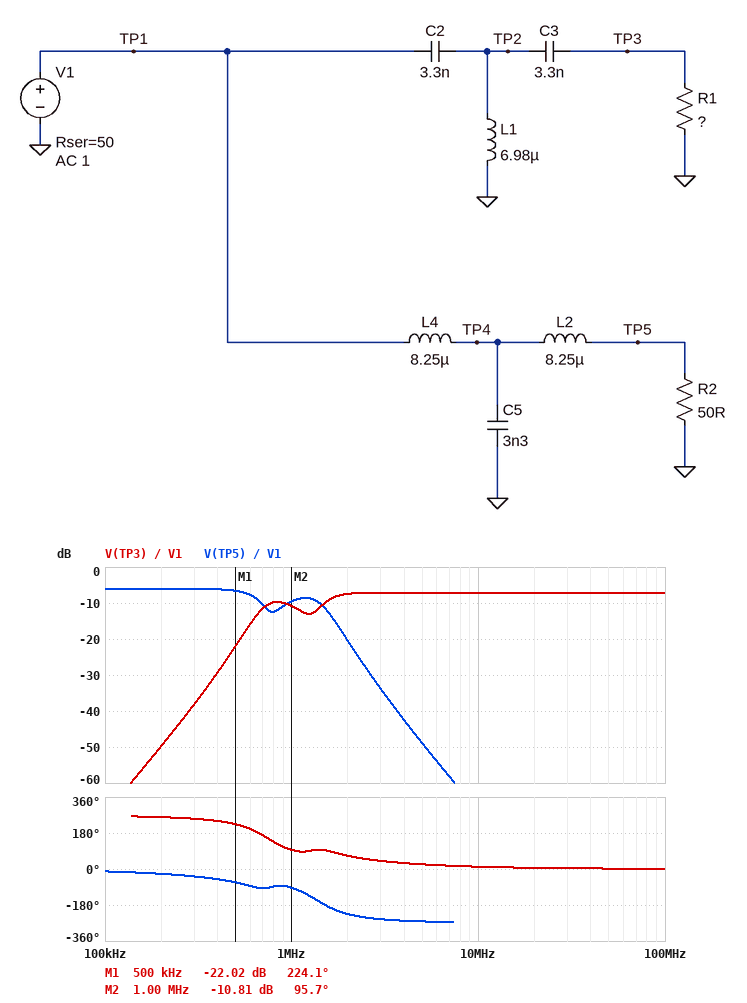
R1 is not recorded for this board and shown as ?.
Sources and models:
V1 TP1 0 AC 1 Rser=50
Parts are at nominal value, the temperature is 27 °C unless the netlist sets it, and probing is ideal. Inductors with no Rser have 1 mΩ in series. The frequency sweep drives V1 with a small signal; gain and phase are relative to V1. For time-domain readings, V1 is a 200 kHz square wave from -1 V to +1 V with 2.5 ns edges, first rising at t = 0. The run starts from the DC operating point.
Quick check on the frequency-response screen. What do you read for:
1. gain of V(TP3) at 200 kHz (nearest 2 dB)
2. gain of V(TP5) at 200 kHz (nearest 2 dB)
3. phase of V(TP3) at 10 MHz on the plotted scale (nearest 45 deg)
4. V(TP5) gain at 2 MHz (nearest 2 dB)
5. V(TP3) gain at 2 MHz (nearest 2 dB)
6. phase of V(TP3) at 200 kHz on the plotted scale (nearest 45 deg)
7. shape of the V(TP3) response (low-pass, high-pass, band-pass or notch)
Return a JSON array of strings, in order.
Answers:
["-50 dB", "-6 dB", "0 deg", "-20 dB", "-8 dB", "270 deg", "high-pass"]
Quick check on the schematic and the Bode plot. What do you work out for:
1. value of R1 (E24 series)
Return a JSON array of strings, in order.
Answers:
["39 Ω"]
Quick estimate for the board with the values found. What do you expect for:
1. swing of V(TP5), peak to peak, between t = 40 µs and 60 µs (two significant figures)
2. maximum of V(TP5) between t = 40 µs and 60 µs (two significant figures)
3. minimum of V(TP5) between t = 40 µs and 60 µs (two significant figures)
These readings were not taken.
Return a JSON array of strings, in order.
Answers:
["1.2 V", "600 mV", "-600 mV"]
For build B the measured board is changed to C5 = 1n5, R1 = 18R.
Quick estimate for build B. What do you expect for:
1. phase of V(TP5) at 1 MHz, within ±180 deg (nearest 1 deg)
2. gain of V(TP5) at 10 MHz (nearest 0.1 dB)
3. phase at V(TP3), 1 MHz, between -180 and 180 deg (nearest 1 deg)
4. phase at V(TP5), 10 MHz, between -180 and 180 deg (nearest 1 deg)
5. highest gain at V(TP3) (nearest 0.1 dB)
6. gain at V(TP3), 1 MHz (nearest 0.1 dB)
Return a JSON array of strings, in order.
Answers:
["-63 deg", "-64.3 dB", "102 deg", "79 deg", "-11.0 dB", "-13.1 dB"]
